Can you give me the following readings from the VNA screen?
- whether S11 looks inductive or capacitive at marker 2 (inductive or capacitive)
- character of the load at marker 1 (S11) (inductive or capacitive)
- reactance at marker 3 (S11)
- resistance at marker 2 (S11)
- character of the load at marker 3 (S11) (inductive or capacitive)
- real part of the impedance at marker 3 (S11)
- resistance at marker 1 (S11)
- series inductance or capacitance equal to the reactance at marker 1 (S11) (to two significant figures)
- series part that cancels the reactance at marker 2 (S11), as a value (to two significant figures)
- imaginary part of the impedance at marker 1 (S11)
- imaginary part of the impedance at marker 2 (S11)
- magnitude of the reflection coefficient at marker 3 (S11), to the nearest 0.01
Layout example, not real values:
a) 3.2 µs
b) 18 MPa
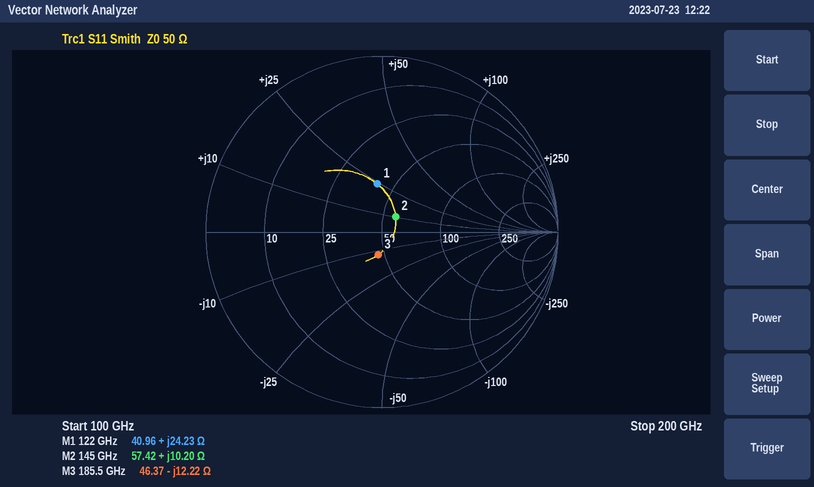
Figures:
a) inductive
b) inductive
c) -12.22 Ω
d) 57.42 Ω
e) capacitive
f) 46.37 Ω
g) 40.96 Ω
h) 32 pH
i) 110 fF
j) +24.23 Ω
k) +10.20 Ω
l) 0.13
